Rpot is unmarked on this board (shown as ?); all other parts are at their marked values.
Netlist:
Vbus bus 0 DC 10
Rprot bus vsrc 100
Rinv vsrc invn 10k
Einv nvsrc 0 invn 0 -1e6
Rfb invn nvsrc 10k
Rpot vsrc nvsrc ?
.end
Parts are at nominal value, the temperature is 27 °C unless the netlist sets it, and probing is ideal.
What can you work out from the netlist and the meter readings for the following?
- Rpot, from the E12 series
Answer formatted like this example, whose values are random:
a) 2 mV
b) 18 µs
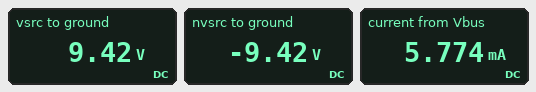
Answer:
a) 3.9 kΩ
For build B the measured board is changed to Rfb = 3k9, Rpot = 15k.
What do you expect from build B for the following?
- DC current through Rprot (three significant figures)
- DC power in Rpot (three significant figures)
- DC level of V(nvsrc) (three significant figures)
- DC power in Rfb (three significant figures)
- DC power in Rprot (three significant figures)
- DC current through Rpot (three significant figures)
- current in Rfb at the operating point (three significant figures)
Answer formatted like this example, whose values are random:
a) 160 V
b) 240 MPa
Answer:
a) 1.89 mA
b) 12.4 mW
c) -3.83 V
d) 3.75 mW
e) 357 µW
f) 909 µA
g) 981 µA
